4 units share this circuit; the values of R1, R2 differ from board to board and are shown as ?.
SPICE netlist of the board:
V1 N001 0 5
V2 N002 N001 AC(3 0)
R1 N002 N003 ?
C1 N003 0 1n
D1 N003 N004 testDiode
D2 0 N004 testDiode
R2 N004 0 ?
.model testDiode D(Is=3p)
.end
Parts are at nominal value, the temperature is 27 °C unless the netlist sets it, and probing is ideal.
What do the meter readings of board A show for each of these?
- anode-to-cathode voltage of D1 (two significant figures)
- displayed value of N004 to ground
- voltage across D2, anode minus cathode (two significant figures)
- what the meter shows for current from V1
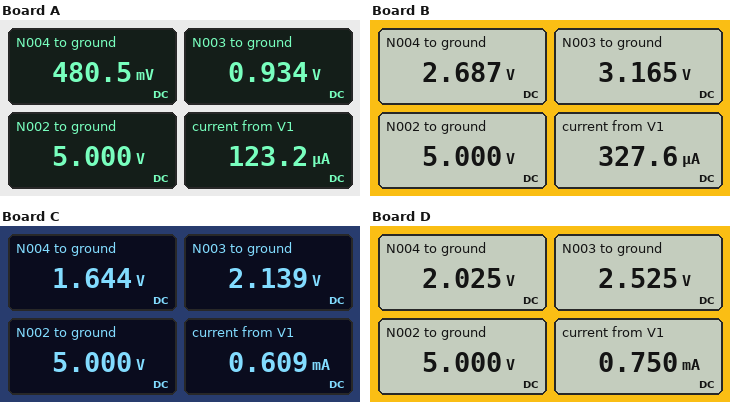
450 mV
480.5 mV
-480 mV
123.2 µA
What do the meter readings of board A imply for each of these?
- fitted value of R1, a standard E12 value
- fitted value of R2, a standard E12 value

33 kΩ
3.9 kΩ
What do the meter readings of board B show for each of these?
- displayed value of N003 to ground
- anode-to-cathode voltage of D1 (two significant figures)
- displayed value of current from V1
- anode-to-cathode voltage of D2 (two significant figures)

3.165 V
480 mV
327.6 µA
-2.7 V
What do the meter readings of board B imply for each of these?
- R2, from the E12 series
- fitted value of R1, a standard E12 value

8.2 kΩ
5.6 kΩ
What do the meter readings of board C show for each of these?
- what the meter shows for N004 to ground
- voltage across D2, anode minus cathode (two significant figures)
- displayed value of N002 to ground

1.644 V
-1.6 V
5.000 V
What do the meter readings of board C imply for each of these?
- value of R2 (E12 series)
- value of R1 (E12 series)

2.7 kΩ
4.7 kΩ
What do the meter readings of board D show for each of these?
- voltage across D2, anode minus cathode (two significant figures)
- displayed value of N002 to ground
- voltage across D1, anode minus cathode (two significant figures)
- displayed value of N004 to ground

-2.0 V
5.000 V
500 mV
2.025 V
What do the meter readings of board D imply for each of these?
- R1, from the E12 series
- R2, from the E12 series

3.3 kΩ
2.7 kΩ
